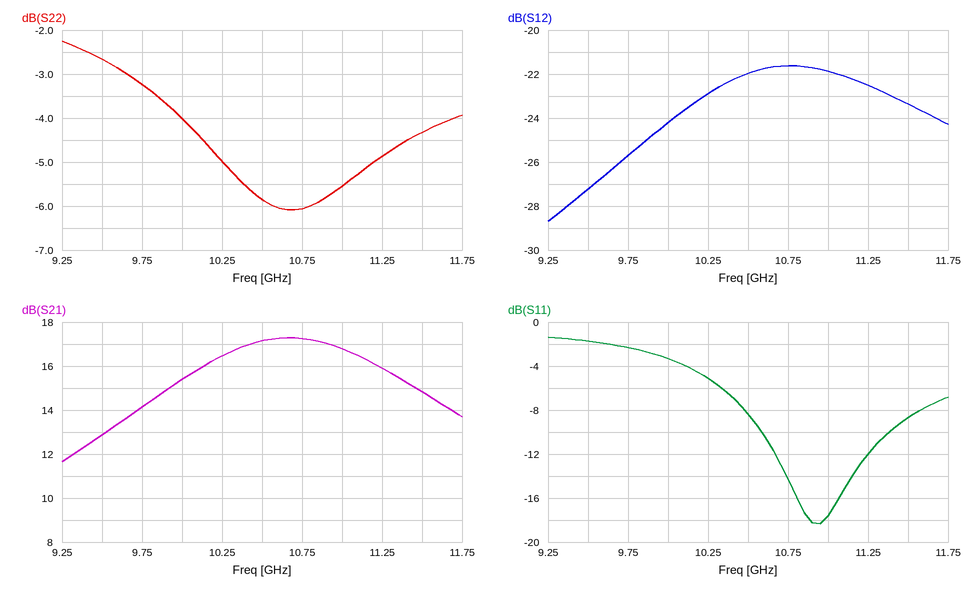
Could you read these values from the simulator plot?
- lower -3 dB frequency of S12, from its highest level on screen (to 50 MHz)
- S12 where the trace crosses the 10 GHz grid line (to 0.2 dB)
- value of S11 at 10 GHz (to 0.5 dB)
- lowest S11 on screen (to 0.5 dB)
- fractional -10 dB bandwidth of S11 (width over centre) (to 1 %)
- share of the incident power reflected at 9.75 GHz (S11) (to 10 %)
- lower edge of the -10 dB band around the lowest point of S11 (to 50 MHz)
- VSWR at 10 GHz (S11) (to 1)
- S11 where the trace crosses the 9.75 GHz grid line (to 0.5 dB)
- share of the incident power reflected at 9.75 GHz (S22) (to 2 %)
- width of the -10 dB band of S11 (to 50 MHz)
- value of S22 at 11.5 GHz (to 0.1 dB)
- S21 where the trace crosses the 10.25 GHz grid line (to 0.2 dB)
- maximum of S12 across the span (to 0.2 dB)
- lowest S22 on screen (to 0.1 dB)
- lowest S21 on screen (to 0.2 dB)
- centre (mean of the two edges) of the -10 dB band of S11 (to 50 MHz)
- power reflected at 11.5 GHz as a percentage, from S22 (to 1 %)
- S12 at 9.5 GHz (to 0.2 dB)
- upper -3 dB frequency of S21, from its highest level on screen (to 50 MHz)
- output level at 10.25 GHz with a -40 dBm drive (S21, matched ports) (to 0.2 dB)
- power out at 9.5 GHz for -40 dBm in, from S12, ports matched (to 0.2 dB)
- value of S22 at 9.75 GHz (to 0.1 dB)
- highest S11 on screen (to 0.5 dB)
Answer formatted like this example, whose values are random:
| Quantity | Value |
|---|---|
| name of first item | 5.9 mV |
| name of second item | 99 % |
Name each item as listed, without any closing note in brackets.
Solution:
| Quantity | Value |
|---|---|
| lower -3 dB frequency of S12, from its highest level on screen | 9.95 GHz |
| S12 where the trace crosses the 10 GHz grid line | -24.2 dB |
| value of S11 at 10 GHz | -3.5 dB |
| lowest S11 on screen | -18.5 dB |
| fractional -10 dB bandwidth of S11 (width over centre) | 7 % |
| share of the incident power reflected at 9.75 GHz (S11) | 60 % |
| lower edge of the -10 dB band around the lowest point of S11 | 10.60 GHz |
| VSWR at 10 GHz (S11) | 5 |
| S11 where the trace crosses the 9.75 GHz grid line | -2.5 dB |
| share of the incident power reflected at 9.75 GHz (S22) | 48 % |
| width of the -10 dB band of S11 | 800 MHz |
| value of S22 at 11.5 GHz | -4.3 dB |
| S21 where the trace crosses the 10.25 GHz grid line | 16.4 dB |
| maximum of S12 across the span | -21.6 dB |
| lowest S22 on screen | -6.1 dB |
| lowest S21 on screen | 11.6 dB |
| centre (mean of the two edges) of the -10 dB band of S11 | 11.00 GHz |
| power reflected at 11.5 GHz as a percentage, from S22 | 37 % |
| S12 at 9.5 GHz | -27.2 dB |
| upper -3 dB frequency of S21, from its highest level on screen | 11.60 GHz |
| output level at 10.25 GHz with a -40 dBm drive (S21, matched ports) | -23.6 dBm |
| power out at 9.5 GHz for -40 dBm in, from S12, ports matched | -67.2 dBm |
| value of S22 at 9.75 GHz | -3.2 dB |
| highest S11 on screen | -1.5 dB |
